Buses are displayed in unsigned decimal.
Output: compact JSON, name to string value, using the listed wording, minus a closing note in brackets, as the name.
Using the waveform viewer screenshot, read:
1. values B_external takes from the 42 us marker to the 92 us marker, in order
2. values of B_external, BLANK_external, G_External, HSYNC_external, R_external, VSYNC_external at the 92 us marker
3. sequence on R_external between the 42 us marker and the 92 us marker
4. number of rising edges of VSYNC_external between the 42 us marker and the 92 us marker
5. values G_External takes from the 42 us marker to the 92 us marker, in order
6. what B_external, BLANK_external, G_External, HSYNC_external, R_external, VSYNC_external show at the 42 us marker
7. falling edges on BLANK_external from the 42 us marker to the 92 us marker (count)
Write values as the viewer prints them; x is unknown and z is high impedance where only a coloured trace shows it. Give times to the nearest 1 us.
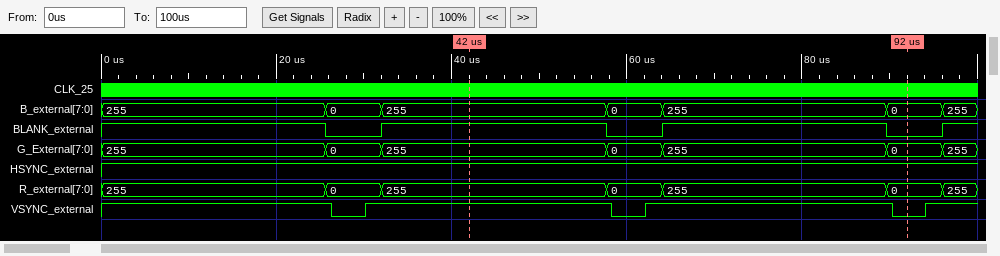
{"values B_external takes from the 42 us marker to the 92 us marker, in order": "255, 0, 255, 0", "values of B_external, BLANK_external, G_External, HSYNC_external, R_external, VSYNC_external at the 92 us marker": "B_external=0, BLANK_external=0, G_External=0, HSYNC_external=1, R_external=0, VSYNC_external=0", "sequence on R_external between the 42 us marker and the 92 us marker": "255, 0, 255, 0", "number of rising edges of VSYNC_external between the 42 us marker and the 92 us marker": "1", "values G_External takes from the 42 us marker to the 92 us marker, in order": "255, 0, 255, 0", "what B_external, BLANK_external, G_External, HSYNC_external, R_external, VSYNC_external show at the 42 us marker": "B_external=255, BLANK_external=1, G_External=255, HSYNC_external=1, R_external=255, VSYNC_external=1", "falling edges on BLANK_external from the 42 us marker to the 92 us marker": "2"}
